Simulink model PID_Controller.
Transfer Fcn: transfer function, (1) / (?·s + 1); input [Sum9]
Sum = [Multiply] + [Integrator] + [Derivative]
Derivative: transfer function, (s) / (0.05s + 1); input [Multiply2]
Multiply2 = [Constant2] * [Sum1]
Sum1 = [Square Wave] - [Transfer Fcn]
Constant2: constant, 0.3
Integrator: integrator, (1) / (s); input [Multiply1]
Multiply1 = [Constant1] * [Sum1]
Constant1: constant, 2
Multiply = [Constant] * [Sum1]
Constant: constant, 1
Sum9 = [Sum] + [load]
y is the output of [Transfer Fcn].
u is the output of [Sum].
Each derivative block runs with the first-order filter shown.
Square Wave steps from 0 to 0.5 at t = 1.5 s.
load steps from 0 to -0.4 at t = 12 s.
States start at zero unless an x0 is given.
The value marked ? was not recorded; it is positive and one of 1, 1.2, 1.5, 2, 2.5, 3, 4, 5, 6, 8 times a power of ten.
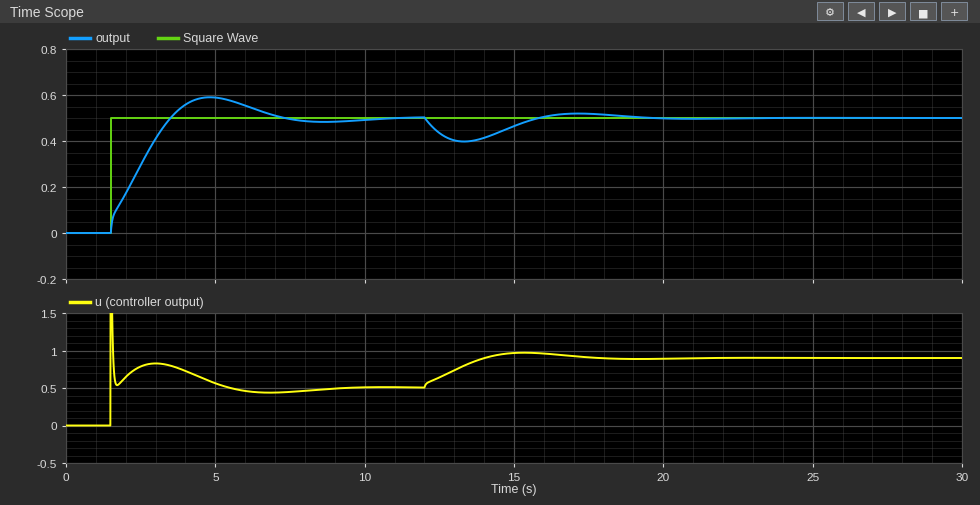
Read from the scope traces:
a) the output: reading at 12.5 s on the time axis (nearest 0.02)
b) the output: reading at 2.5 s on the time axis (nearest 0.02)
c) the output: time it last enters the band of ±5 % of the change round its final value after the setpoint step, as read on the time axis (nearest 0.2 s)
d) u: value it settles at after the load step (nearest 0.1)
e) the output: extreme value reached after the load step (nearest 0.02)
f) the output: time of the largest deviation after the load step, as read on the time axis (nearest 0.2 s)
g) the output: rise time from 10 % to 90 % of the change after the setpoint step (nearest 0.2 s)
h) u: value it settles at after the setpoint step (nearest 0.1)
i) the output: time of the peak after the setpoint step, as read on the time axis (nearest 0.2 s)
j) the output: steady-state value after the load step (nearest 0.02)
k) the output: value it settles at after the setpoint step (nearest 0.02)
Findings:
0.44
0.30
6.6 s
0.9
0.40
13.4 s
1.6 s
0.5
4.8 s
0.50
0.50
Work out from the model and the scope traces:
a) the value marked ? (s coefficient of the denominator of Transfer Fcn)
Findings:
2
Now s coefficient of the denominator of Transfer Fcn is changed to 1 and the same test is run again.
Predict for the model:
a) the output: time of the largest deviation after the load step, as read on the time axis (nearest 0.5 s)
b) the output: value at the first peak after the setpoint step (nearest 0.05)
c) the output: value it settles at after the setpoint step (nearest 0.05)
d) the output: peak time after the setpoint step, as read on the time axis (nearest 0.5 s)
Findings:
13.0 s
0.55
0.50
4.5 s
